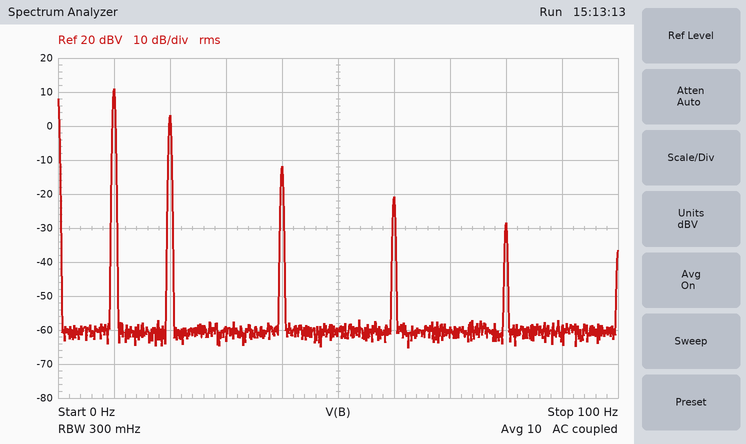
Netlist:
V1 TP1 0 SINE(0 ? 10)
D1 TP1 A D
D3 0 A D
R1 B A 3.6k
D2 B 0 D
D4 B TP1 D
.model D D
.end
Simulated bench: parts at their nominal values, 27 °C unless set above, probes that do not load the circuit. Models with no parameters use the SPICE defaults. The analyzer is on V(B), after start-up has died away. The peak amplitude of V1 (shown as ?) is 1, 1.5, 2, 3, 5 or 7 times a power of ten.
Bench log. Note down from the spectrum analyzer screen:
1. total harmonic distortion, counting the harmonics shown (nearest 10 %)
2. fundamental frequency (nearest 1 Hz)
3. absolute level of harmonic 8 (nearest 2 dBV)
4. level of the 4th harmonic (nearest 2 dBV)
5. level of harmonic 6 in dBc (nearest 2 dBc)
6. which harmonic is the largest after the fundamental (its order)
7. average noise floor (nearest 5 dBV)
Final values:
40 %
10 Hz
-28 dBV
-12 dBV
-32 dBc
2
-60 dBV
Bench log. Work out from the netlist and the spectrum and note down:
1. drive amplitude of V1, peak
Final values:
10 V
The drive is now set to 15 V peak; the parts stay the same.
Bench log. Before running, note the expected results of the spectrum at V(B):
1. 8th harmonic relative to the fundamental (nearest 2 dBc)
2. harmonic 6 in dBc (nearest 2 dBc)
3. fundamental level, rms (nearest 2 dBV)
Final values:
-36 dBc
-30 dBc
14 dBV
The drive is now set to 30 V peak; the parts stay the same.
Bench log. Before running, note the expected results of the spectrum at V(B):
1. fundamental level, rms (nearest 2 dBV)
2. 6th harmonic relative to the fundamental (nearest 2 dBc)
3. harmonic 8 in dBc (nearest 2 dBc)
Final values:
20 dBV
-30 dBc
-34 dBc
